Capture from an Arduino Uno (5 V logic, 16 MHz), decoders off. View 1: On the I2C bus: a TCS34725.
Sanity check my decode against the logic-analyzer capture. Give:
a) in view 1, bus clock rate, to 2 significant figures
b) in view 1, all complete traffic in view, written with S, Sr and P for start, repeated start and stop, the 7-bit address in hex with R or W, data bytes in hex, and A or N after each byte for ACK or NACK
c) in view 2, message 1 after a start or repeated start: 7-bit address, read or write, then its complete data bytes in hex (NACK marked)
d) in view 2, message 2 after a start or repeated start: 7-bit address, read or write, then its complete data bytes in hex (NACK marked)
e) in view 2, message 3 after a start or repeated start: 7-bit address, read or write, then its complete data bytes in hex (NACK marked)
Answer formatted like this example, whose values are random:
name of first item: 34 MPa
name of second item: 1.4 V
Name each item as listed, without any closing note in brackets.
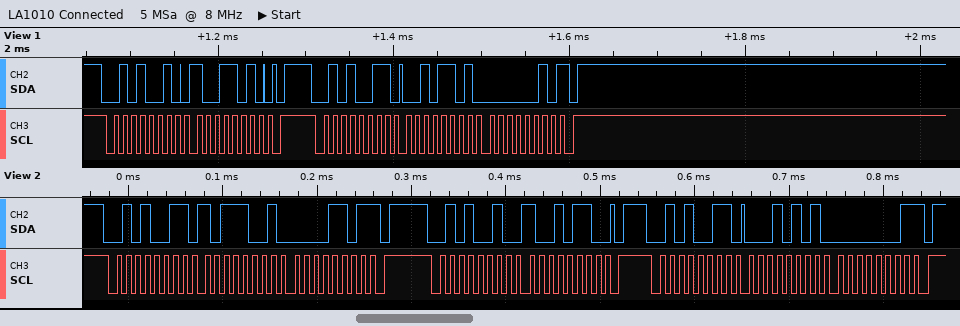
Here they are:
in view 1, bus clock rate, to 2 significant figures: 100 kHz
in view 1, all complete traffic in view, written with S, Sr and P for start, repeated start and stop, the 7-bit address in hex with R or W, data bytes in hex, and A or N after each byte for ACK or NACK: S 29W A 9A A P S 29R A 2D A 02 N P
in view 2, message 1 after a start or repeated start: 7-bit address, read or write, then its complete data bytes in hex: 0x29 read: B9 0D NACK
in view 2, message 2 after a start or repeated start: 7-bit address, read or write, then its complete data bytes in hex: 0x29 write: 96
in view 2, message 3 after a start or repeated start: 7-bit address, read or write, then its complete data bytes in hex: 0x29 read: 15 01 NACK
